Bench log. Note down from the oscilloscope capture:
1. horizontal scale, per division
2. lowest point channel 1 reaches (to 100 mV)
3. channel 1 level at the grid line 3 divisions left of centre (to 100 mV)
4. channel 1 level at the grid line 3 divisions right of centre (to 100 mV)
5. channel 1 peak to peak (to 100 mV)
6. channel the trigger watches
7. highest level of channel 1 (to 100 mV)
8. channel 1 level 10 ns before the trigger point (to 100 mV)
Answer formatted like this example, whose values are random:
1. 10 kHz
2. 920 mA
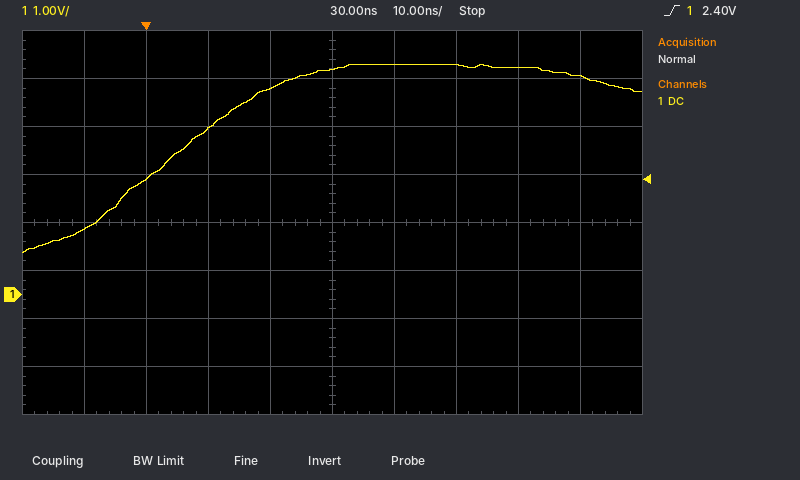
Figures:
1. 10 ns
2. 900 mV
3. 2.4 V
4. 4.7 V
5. 3.9 V
6. channel 1
7. 4.8 V
8. 1.4 V
